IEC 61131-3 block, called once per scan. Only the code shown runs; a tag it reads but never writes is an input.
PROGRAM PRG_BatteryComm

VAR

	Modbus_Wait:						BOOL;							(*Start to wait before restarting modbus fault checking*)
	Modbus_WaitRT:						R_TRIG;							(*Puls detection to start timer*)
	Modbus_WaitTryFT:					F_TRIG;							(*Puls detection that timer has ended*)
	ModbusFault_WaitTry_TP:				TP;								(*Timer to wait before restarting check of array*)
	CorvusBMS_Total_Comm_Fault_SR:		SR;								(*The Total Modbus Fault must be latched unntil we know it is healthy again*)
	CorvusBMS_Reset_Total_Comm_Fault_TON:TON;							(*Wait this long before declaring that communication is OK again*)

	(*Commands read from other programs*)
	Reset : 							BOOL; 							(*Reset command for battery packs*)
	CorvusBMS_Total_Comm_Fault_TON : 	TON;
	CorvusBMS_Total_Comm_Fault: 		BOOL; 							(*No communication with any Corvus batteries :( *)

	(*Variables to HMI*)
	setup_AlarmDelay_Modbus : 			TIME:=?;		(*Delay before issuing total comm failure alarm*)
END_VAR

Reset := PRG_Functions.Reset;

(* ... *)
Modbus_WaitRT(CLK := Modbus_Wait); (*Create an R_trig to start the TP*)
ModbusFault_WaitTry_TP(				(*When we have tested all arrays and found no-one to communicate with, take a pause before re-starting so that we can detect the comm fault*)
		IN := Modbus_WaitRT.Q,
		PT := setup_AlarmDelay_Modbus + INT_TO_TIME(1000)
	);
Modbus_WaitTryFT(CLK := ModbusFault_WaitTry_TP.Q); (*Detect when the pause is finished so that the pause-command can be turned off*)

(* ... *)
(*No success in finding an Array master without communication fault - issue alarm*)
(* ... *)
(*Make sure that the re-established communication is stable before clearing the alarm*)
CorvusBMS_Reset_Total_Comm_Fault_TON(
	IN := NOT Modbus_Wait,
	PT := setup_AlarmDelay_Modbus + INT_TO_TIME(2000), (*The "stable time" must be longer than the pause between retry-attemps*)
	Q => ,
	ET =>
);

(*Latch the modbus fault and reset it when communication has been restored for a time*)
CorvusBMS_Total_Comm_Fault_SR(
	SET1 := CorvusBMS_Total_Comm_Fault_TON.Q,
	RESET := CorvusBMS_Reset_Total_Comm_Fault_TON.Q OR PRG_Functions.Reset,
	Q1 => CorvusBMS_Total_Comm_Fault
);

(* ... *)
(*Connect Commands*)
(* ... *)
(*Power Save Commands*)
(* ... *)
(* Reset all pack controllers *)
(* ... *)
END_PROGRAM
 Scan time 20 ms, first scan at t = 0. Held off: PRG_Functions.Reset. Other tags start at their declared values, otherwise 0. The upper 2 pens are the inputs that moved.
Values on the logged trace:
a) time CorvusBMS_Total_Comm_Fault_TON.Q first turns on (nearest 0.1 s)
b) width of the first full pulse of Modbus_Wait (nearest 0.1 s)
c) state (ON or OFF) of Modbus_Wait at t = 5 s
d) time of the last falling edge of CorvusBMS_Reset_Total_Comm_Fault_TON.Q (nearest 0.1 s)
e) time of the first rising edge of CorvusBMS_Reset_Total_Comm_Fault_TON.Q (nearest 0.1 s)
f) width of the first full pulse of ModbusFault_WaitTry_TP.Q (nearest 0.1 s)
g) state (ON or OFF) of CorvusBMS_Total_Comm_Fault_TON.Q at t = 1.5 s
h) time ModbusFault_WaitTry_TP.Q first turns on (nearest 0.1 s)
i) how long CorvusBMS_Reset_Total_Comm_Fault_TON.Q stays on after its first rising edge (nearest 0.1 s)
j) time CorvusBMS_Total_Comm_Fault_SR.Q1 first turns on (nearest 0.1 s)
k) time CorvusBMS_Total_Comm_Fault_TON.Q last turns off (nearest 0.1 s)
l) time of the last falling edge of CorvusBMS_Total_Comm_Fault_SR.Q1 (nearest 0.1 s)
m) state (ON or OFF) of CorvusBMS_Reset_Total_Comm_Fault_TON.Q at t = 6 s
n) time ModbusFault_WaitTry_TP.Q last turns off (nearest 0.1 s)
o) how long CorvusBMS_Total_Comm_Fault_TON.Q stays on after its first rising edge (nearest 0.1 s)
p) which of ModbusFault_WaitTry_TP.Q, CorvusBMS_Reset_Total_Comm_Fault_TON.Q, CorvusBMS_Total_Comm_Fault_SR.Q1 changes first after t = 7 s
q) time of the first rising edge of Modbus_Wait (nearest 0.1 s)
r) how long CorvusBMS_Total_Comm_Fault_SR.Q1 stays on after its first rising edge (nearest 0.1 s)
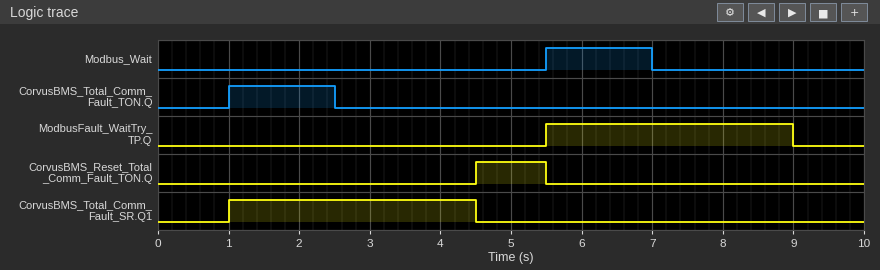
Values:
1.0 s
1.5 s
OFF
5.5 s
4.5 s
3.5 s
ON
5.5 s
1.0 s
1.0 s
2.5 s
4.5 s
OFF
9.0 s
1.5 s
ModbusFault_WaitTry_TP.Q
5.5 s
3.5 s
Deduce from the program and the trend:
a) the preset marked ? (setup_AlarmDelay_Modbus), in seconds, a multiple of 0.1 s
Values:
2.5 s
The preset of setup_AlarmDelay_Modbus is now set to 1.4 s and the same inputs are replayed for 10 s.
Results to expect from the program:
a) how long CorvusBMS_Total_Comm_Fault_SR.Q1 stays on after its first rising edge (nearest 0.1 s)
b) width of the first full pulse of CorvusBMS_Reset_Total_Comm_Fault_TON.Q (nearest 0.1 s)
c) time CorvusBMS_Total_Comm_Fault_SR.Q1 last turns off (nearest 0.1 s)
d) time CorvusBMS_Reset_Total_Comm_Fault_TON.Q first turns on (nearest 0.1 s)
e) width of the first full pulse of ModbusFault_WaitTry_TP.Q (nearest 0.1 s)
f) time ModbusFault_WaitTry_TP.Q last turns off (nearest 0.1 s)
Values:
2.4 s
2.1 s
3.4 s
3.4 s
2.4 s
7.9 s
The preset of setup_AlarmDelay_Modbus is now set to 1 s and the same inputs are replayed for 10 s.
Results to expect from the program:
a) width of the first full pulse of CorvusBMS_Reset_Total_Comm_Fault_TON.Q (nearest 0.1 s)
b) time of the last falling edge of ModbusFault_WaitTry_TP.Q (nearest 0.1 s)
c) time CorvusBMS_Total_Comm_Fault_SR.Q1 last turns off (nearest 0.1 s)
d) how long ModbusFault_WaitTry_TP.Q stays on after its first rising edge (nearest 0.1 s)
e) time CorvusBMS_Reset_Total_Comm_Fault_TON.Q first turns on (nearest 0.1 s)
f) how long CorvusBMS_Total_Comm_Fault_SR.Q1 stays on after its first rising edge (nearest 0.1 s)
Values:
2.5 s
7.5 s
3.0 s
2.0 s
3.0 s
2.0 s
